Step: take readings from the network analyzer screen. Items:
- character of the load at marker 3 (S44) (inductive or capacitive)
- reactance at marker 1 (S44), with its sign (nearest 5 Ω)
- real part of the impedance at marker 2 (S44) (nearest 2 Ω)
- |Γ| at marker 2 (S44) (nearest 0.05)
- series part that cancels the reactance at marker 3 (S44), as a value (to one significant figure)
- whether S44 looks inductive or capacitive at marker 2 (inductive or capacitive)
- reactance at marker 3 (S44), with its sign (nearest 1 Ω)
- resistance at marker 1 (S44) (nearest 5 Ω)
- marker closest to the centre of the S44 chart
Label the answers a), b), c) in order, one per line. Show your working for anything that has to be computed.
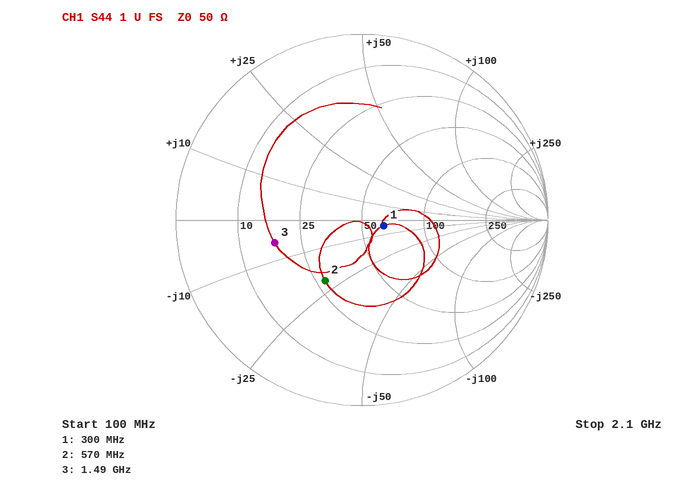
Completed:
a) capacitive
b) -5 Ω
c) 28 Ω
d) 0.40
e) L = 6 Ω/(2π × 1.49 GHz) ≈ 641 pH, so 600 pH to one significant figure
f) capacitive
g) -6 Ω
h) 65 Ω
i) marker 1
